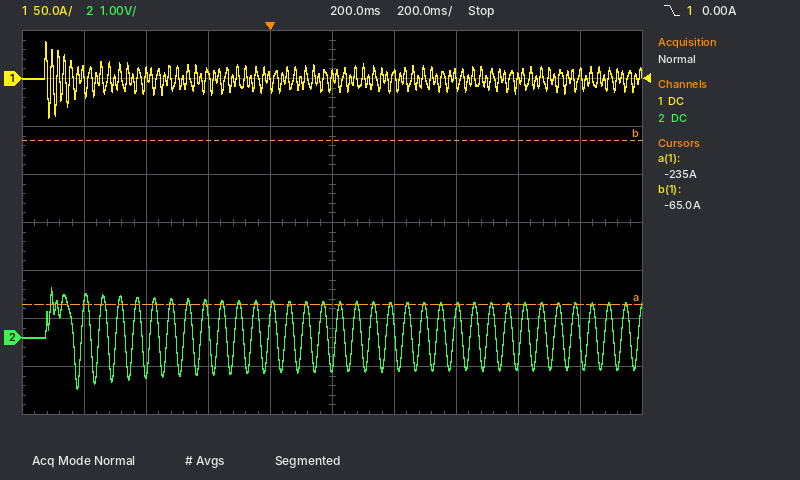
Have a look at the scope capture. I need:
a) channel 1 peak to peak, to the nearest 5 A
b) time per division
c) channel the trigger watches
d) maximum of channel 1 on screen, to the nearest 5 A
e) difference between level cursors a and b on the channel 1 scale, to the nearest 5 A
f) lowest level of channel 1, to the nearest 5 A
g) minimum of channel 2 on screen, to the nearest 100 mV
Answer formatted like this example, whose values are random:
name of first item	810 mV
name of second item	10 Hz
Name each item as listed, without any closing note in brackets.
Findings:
channel 1 peak to peak, to the nearest 5 A	80 A
time per division	200 ms
channel the trigger watches	channel 1
maximum of channel 1 on screen, to the nearest 5 A	40 A
difference between level cursors a and b on the channel 1 scale, to the nearest 5 A	170 A
lowest level of channel 1, to the nearest 5 A	-40 A
minimum of channel 2 on screen, to the nearest 100 mV	-1.1 V
